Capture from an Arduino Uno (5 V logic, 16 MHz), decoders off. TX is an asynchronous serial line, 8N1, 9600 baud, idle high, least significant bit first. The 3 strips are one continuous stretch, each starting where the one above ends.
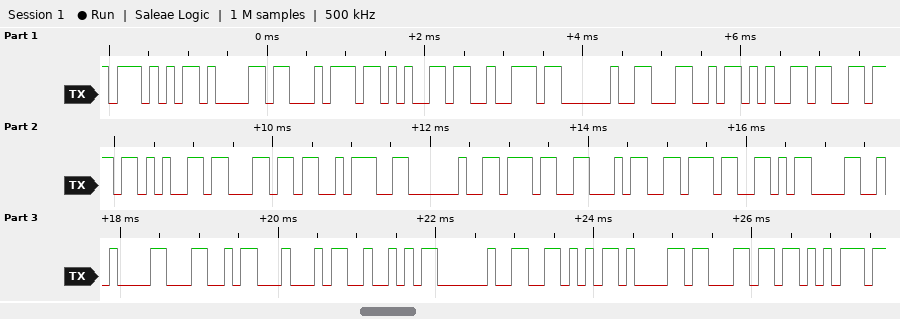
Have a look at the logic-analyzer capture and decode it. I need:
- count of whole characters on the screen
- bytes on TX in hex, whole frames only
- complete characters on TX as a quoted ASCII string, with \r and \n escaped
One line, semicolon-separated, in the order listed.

26; 0x57 0x61 0x74 0x65 0x72 0x20 0x4C 0x65 0x76 0x65 0x6C 0x3A 0x20 0x37 0x34 0x37 0x0D 0x0A 0x4C 0x44 0x52 0x20 0x56 0x61 0x6C 0x75; "Water Level: 747\r\nLDR Valu"
